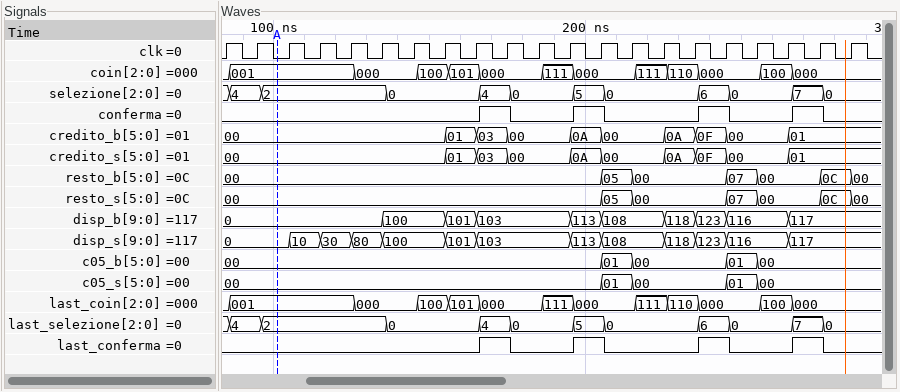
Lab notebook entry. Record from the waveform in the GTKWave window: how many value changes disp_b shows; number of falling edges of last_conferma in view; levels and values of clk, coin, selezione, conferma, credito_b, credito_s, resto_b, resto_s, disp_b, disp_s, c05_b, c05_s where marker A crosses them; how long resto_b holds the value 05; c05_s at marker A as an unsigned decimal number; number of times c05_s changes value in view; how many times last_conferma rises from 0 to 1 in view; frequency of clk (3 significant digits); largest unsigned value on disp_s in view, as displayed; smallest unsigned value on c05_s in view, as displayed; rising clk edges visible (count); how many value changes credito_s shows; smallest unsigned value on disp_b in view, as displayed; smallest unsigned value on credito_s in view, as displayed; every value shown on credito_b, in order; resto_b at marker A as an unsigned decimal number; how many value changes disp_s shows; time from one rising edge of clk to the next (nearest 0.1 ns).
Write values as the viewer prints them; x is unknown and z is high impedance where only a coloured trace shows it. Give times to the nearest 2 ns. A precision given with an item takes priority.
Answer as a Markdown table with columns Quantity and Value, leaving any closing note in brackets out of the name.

| Quantity | Value |
|---|---|
| how many value changes disp_b shows | 9 |
| number of falling edges of last_conferma in view | 4 |
| levels and values of clk, coin, selezione, conferma, credito_b, credito_s, resto_b, resto_s, disp_b, disp_s, c05_b, c05_s where marker A crosses them | clk=0, coin=001, selezione=2, conferma=0, credito_b=00, credito_s=00, resto_b=00, resto_s=00, disp_b=0, disp_s=0, c05_b=00, c05_s=00 |
| how long resto_b holds the value 05 | 10 ns |
| c05_s at marker A as an unsigned decimal number | 0 |
| number of times c05_s changes value in view | 4 |
| how many times last_conferma rises from 0 to 1 in view | 4 |
| frequency of clk | 100 MHz |
| largest unsigned value on disp_s in view, as displayed | 123 |
| smallest unsigned value on c05_s in view, as displayed | 00 |
| rising clk edges visible | 21 |
| how many value changes credito_s shows | 9 |
| smallest unsigned value on disp_b in view, as displayed | 0 |
| smallest unsigned value on credito_s in view, as displayed | 00 |
| every value shown on credito_b, in order | 00, 01, 03, 00, 0A, 00, 0A, 0F, 00, 01 |
| resto_b at marker A as an unsigned decimal number | 0 |
| how many value changes disp_s shows | 12 |
| time from one rising edge of clk to the next | 10 ns |
